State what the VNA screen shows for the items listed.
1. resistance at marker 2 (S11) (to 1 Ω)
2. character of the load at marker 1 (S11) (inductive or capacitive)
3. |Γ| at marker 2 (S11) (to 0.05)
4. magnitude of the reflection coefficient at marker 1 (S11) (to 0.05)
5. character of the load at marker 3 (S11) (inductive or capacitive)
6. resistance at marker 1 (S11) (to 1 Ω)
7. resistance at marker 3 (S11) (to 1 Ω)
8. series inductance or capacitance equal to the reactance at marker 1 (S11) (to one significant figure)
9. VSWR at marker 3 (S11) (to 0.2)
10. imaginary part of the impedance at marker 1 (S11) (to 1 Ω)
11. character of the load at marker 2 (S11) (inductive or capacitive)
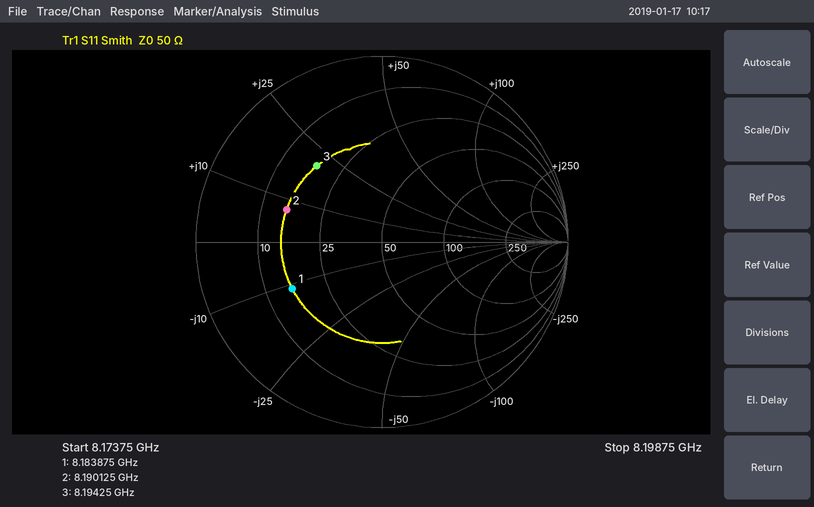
15 Ω
capacitive
0.55
0.55
inductive
16 Ω
18 Ω
2 pF
3.4
-11 Ω
inductive
